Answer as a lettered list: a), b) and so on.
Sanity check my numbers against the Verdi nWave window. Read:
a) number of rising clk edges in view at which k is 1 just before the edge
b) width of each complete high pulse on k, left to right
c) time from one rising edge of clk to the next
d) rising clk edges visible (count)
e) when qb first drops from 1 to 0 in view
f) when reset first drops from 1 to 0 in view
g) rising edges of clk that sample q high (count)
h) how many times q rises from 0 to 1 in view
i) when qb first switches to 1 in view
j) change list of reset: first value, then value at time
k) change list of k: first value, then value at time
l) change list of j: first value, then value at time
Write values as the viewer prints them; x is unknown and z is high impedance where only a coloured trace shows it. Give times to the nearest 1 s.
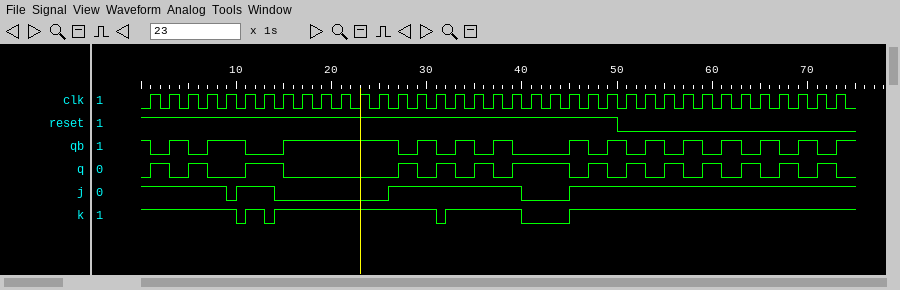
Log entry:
a) 33
b) 2 s, 17 s, 8 s
c) 2 s
d) 37
e) 1 s
f) 50 s
g) 17
h) 14
i) 3 s
j) 1, 0 at 50 s
k) 1, 0 at 10 s, 1 at 11 s, 0 at 13 s, 1 at 14 s, 0 at 31 s, 1 at 32 s, 0 at 40 s, 1 at 45 s
l) 1, 0 at 9 s, 1 at 10 s, 0 at 14 s, 1 at 26 s, 0 at 40 s, 1 at 45 s
